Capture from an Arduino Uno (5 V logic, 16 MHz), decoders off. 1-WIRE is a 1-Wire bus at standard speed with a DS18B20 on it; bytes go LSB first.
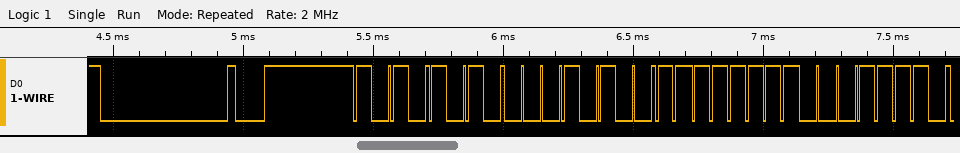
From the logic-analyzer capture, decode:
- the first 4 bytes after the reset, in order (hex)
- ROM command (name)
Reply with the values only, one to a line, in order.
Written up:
55 28 FF 78
Match ROM
